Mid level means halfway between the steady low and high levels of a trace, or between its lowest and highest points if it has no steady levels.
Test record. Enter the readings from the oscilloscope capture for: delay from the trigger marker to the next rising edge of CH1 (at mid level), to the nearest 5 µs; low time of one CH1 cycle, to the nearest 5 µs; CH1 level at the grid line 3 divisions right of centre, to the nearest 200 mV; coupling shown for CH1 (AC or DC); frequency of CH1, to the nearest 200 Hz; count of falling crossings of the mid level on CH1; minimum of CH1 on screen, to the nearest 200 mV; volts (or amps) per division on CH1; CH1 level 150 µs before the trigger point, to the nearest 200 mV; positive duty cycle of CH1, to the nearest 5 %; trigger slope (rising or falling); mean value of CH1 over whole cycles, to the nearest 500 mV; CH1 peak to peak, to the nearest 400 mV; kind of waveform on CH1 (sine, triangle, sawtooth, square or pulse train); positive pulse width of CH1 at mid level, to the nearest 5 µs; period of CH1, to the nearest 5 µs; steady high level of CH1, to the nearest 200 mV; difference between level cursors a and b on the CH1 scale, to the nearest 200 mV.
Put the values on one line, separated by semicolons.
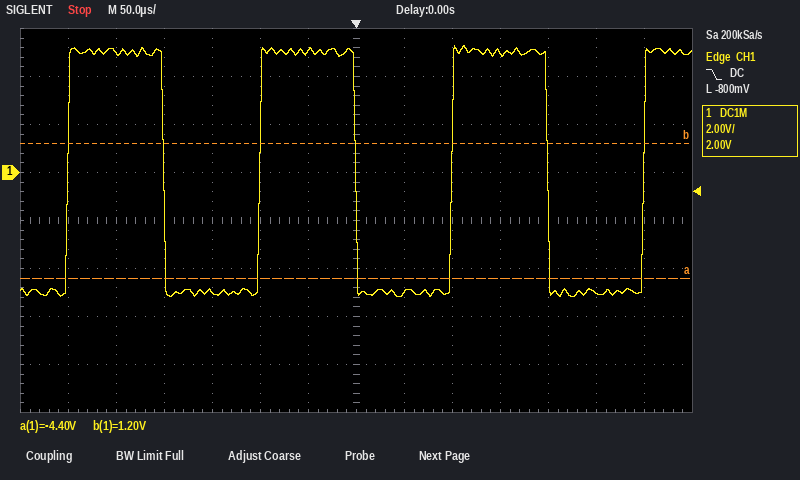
100 µs; 100 µs; 5.0 V; DC; 5.0 kHz; 3; -5.2 V; 2 V; -5.0 V; 50 %; falling; 0.0 V; 10.4 V; square; 100 µs; 200 µs; 5.0 V; 5.6 V
